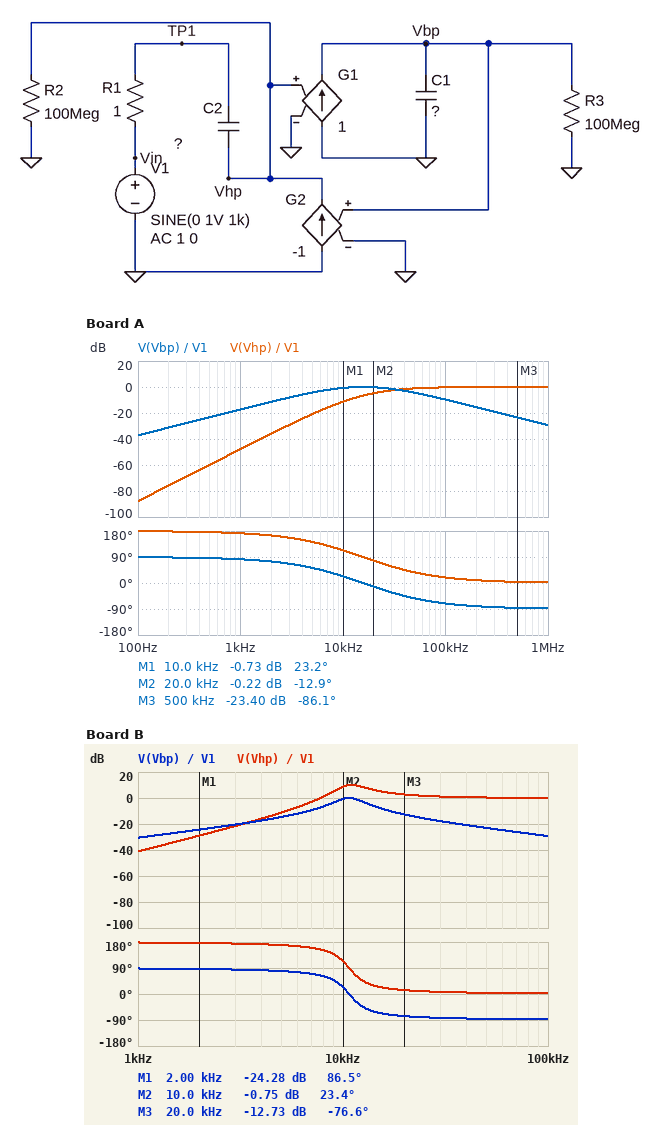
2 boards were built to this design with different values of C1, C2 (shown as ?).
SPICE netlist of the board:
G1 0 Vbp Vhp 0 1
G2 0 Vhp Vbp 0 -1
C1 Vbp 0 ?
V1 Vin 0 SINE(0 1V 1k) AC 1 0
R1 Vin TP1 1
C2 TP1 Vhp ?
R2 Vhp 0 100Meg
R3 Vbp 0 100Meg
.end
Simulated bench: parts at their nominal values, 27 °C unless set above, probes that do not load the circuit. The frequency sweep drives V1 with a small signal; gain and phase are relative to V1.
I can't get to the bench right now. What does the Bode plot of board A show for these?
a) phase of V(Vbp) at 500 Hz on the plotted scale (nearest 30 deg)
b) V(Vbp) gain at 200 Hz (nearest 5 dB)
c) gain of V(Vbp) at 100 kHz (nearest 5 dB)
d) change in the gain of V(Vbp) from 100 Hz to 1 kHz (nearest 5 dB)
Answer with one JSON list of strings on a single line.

["90 deg", "-30 dB", "-10 dB", "20 dB"]
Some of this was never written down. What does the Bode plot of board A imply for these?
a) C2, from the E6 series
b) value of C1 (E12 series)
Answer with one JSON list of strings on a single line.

["22 µF", "4.7 µF"]
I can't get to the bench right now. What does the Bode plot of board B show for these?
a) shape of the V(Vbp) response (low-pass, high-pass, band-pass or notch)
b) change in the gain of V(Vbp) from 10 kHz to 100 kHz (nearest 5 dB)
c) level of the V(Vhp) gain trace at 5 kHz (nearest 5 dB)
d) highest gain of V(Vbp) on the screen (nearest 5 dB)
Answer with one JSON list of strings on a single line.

["band-pass", "-30 dB", "-10 dB", "0 dB"]
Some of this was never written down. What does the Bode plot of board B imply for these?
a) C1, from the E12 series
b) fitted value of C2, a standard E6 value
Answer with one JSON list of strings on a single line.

["47 µF", "4.7 µF"]
